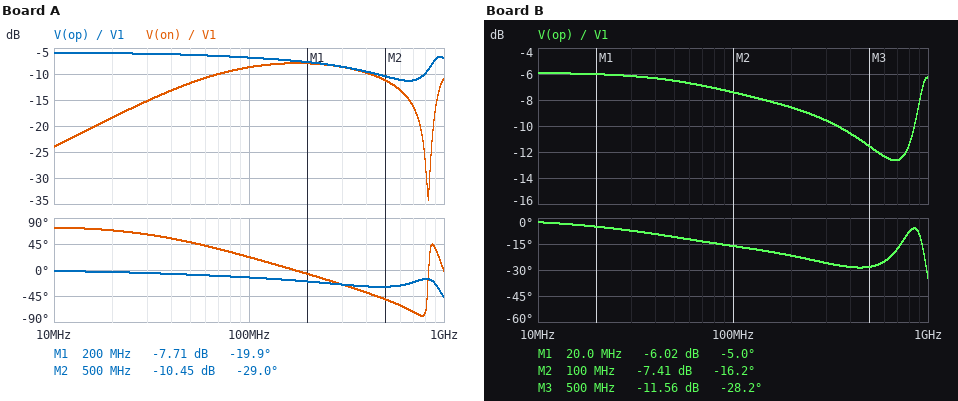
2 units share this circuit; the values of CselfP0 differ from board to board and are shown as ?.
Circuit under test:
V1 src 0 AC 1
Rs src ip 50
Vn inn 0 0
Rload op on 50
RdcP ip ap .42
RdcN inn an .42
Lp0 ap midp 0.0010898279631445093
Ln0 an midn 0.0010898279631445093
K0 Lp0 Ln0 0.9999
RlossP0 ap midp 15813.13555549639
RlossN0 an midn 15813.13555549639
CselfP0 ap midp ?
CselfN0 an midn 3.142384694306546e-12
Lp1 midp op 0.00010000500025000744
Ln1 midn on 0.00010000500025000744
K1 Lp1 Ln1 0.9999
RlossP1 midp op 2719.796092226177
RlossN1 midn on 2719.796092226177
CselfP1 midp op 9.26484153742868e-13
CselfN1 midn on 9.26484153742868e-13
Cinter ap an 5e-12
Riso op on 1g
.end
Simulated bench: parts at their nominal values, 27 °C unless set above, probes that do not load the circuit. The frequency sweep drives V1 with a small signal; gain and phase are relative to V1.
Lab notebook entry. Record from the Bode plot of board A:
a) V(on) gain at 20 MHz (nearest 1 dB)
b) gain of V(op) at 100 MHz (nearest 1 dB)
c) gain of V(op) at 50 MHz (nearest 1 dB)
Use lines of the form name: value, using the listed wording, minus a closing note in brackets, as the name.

V(on) gain at 20 MHz: -18 dB
gain of V(op) at 100 MHz: -7 dB
gain of V(op) at 50 MHz: -6 dB
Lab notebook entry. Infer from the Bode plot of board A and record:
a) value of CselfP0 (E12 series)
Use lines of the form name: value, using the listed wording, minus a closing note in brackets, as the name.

value of CselfP0: 2.2 pF
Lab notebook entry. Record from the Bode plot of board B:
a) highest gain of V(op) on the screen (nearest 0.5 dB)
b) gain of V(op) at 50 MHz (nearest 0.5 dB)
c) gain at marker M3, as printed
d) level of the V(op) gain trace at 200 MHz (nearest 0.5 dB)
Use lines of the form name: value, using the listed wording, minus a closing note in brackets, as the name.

highest gain of V(op) on the screen: -6.0 dB
gain of V(op) at 50 MHz: -6.5 dB
gain at marker M3, as printed: -11.56 dB
level of the V(op) gain trace at 200 MHz: -8.5 dB
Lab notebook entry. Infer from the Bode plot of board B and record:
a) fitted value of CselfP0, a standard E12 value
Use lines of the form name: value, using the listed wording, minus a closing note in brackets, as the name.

fitted value of CselfP0, a standard E12 value: 1.8 pF
